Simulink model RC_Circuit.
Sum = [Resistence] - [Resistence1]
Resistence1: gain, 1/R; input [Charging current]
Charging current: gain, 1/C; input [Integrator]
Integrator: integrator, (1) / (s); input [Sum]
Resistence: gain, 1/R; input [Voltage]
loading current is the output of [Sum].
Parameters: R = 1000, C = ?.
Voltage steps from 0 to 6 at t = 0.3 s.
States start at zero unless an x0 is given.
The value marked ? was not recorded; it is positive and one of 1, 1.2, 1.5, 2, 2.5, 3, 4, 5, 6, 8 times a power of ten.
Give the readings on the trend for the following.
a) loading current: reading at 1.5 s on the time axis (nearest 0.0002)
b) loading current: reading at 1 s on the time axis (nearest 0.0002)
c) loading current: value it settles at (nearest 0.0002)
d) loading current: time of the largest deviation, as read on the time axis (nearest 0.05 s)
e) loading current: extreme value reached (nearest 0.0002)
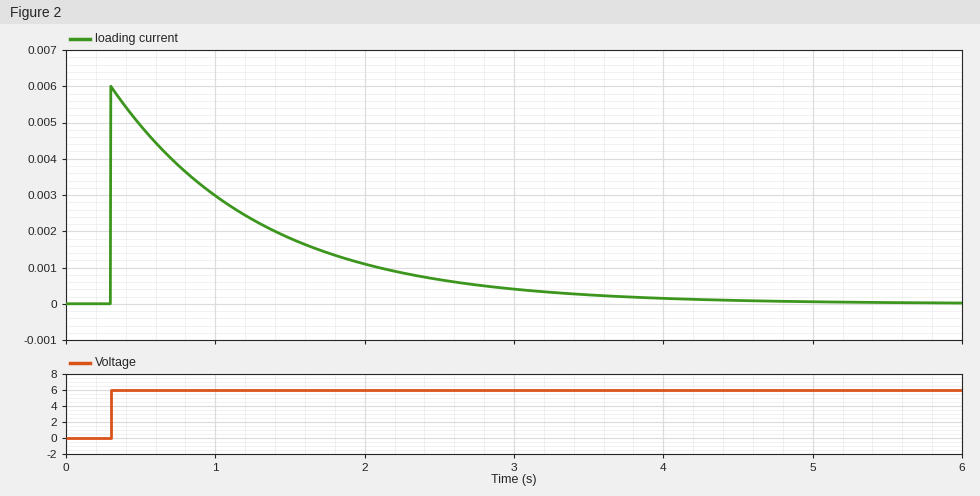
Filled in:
0.0018
0.0030
0.0000
0.30 s
0.0060
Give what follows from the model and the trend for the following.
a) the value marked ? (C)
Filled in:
0.001
